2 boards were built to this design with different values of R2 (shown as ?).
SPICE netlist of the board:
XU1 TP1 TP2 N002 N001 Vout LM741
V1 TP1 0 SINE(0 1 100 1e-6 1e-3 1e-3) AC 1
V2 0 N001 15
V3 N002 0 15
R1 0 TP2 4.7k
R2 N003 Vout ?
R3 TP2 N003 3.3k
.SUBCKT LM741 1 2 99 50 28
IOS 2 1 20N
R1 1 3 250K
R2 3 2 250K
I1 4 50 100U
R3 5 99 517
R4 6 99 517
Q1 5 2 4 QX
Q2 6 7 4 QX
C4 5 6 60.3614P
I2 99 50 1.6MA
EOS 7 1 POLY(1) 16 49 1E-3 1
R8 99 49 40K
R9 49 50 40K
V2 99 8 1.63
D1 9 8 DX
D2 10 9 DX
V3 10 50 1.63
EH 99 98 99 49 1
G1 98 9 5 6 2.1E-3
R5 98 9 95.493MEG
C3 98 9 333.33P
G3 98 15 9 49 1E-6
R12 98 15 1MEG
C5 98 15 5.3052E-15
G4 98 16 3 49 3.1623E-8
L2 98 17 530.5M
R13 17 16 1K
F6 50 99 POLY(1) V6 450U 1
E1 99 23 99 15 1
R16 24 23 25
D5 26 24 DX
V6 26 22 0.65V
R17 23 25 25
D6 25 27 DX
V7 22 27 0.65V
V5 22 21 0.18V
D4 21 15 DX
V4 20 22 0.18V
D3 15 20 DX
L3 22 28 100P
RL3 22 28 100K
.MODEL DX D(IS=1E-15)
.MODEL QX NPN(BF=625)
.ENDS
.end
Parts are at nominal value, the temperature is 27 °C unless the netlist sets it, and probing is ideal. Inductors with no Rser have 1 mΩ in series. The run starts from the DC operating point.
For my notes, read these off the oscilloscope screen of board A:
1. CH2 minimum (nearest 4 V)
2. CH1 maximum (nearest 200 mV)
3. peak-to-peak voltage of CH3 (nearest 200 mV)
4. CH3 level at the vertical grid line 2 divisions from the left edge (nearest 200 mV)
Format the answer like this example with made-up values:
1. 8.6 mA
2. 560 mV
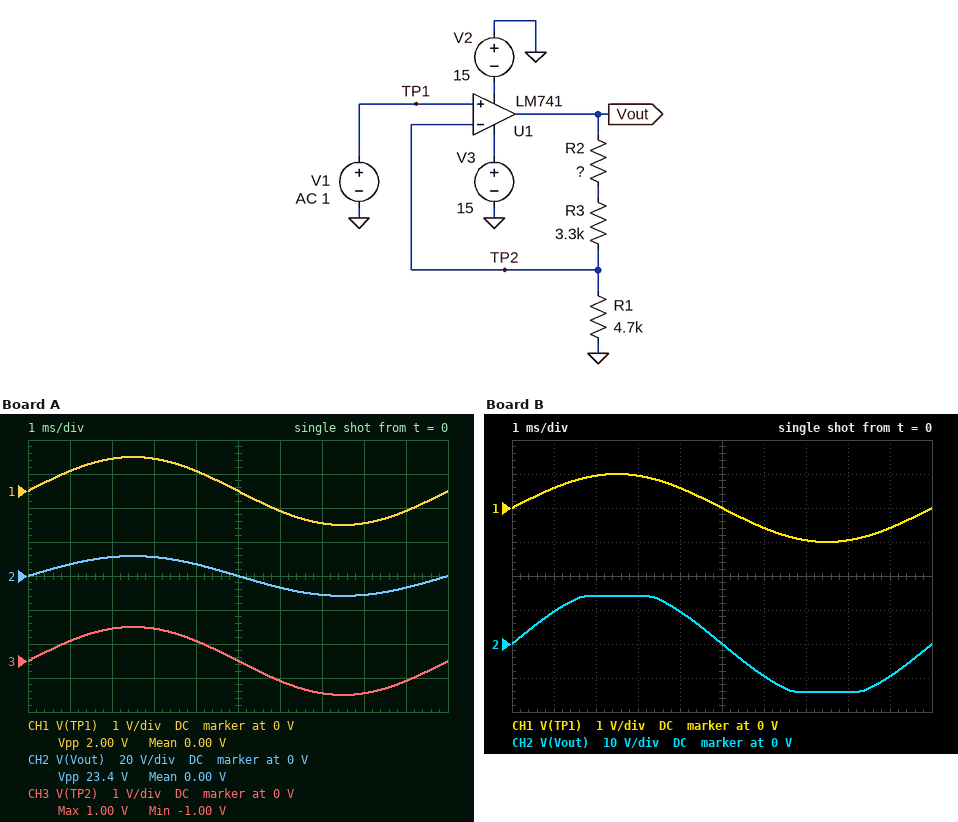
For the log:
1. -12 V
2. 1.0 V
3. 2.0 V
4. 1.0 V
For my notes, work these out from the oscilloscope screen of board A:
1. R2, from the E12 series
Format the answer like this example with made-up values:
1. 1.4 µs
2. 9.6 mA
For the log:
1. 47 kΩ
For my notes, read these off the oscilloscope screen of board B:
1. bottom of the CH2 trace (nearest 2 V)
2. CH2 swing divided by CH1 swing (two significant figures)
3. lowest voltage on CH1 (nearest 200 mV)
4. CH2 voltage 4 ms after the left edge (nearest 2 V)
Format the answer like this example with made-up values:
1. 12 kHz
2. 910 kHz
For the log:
1. -14 V
2. 14
3. -1.0 V
4. 10 V
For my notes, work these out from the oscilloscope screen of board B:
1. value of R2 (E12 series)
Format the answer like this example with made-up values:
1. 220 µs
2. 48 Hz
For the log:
1. 68 kΩ
